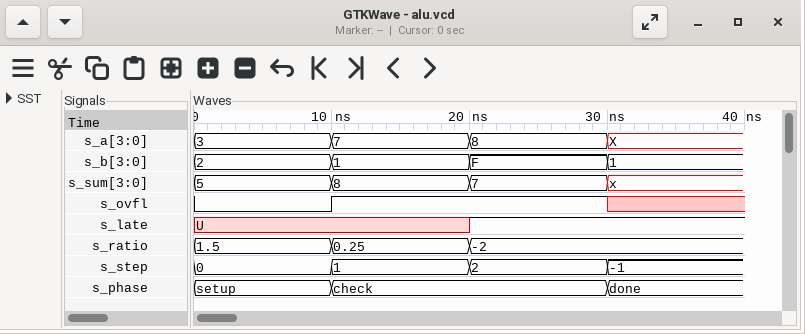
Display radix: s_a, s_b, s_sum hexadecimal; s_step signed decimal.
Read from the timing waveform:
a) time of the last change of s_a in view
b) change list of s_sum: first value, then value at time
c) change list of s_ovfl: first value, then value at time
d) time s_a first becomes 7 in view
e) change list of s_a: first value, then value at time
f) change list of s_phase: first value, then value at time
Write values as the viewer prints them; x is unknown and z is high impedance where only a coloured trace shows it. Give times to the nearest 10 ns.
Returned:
30 ns
5, 8 at 10 ns, 7 at 20 ns, x at 30 ns
0, 1 at 10 ns, x at 30 ns
10 ns
3, 7 at 10 ns, 8 at 20 ns, X at 30 ns
setup, check at 10 ns, done at 30 ns
